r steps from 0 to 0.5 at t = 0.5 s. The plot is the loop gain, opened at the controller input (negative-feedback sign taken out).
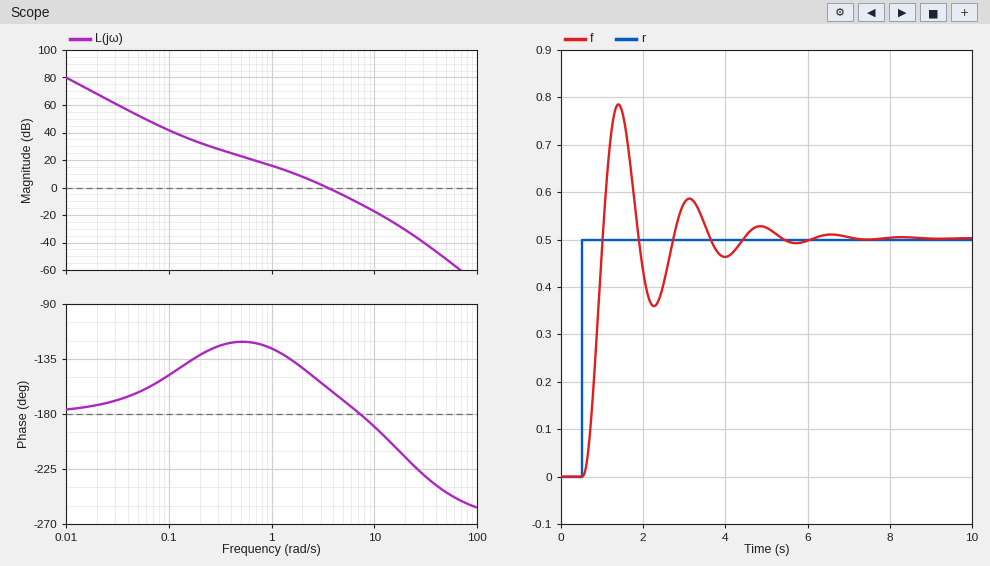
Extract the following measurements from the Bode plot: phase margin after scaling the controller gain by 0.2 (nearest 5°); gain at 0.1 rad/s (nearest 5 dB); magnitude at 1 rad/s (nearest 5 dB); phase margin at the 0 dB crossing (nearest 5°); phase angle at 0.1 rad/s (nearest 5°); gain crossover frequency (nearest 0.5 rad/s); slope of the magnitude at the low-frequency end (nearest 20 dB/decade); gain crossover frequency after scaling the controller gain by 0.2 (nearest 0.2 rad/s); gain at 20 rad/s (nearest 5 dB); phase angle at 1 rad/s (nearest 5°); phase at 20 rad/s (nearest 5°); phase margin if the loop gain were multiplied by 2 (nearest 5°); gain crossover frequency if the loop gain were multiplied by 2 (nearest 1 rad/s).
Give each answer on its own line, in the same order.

50°
40 dB
15 dB
20°
-150°
3.5 rad/s
-40 dB/decade
1.2 rad/s
-30 dB
-125°
-215°
10°
5 rad/s
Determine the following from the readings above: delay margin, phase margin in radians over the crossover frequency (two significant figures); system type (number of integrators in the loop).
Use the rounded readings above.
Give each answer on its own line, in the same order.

0.100 s
2
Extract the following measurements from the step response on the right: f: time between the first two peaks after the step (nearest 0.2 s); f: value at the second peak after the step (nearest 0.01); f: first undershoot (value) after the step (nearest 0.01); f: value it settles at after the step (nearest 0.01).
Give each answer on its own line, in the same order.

1.8 s
0.59
0.36
0.50
